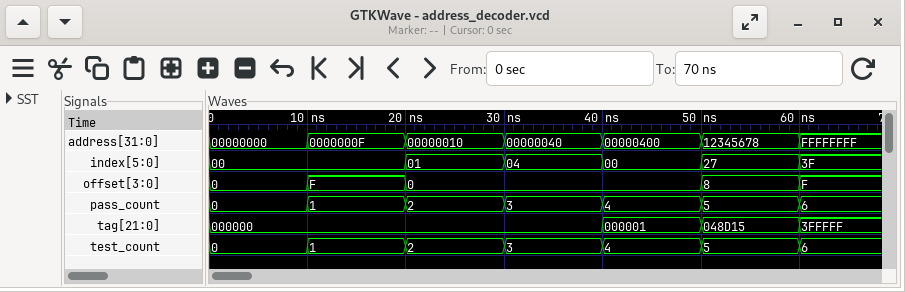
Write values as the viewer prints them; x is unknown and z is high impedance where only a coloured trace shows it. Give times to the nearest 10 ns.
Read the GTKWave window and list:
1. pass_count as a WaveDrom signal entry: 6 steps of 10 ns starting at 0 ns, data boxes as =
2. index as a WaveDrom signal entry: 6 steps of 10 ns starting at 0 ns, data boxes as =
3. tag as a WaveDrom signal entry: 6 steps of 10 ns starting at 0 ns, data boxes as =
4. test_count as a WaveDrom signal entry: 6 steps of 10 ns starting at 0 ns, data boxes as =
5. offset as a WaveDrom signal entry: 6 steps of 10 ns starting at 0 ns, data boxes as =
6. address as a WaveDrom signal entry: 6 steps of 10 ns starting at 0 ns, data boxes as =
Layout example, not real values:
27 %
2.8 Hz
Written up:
{name: 'pass_count', wave: '======', data: '0 1 2 3 4 5'}
{name: 'index', wave: '=.====', data: '00 01 04 00 27'}
{name: 'tag', wave: '=...==', data: '000000 000001 048D15'}
{name: 'test_count', wave: '======', data: '0 1 2 3 4 5'}
{name: 'offset', wave: '===..=', data: '0 F 0 8'}
{name: 'address', wave: '======', data: '00000000 0000000F 00000010 00000040 00000400 12345678'}
